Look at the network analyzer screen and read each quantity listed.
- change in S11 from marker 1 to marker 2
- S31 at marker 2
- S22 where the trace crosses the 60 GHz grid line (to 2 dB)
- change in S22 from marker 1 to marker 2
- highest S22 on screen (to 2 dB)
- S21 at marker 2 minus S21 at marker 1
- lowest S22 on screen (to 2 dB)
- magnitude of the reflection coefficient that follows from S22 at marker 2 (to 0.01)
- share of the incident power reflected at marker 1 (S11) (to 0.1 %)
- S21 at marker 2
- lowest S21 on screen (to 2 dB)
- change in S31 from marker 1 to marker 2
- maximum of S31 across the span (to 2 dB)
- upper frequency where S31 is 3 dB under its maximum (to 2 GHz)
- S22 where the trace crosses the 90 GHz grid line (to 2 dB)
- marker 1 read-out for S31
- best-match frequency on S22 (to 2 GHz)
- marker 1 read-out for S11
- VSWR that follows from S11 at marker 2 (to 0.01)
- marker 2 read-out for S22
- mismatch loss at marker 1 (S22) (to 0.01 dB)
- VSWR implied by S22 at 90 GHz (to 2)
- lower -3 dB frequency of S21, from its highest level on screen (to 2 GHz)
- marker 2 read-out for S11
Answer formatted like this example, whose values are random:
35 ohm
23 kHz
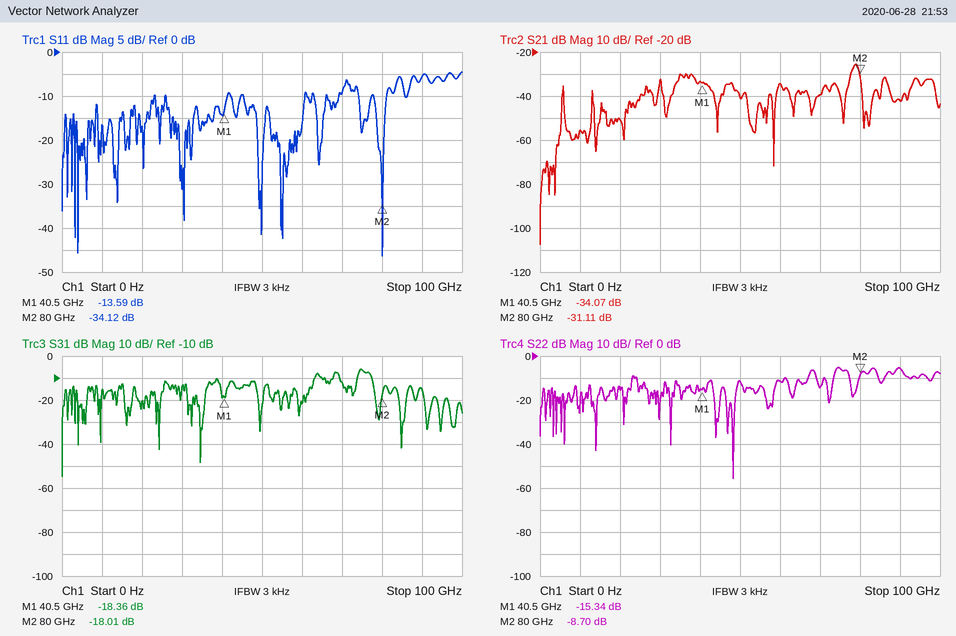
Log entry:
-20.53 dB
-18.01 dB
-12 dB
6.64 dB
-6 dB
2.96 dB
-56 dB
0.37
4.4 %
-31.11 dB
-108 dB
0.35 dB
-6 dB
78 GHz
-6 dB
-18.36 dB
48 GHz
-13.59 dB
1.04
-8.70 dB
0.13 dB
4
78 GHz
-34.12 dB
